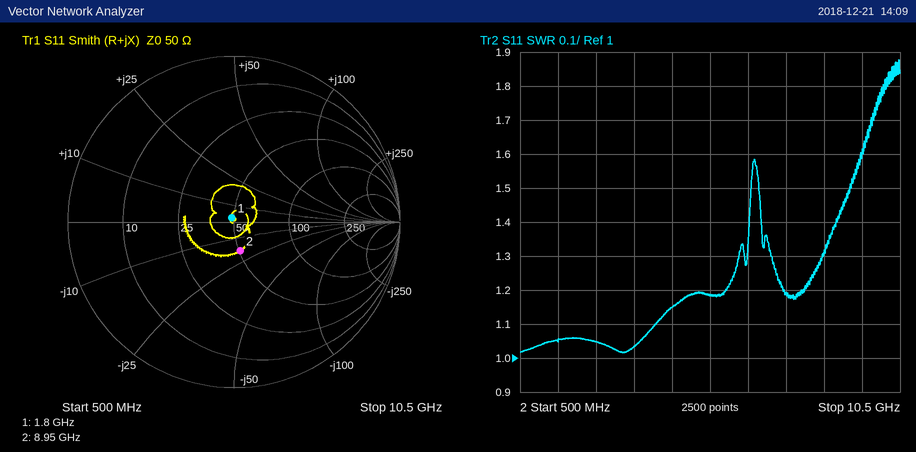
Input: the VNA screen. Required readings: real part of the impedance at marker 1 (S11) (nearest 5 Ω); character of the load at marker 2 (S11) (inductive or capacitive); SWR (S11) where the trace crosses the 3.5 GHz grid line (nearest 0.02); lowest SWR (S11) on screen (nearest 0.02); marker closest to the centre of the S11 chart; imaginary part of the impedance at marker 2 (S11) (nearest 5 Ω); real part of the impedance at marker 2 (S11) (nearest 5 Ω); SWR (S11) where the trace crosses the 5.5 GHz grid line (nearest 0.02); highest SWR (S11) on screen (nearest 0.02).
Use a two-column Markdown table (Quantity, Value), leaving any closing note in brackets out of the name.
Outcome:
| Quantity | Value |
|---|---|
| real part of the impedance at marker 1 (S11) | 50 Ω |
| character of the load at marker 2 (S11) | capacitive |
| SWR (S11) where the trace crosses the 3.5 GHz grid line | 1.04 |
| lowest SWR (S11) on screen | 1.02 |
| marker closest to the centre of the S11 chart | marker 1 |
| imaginary part of the impedance at marker 2 (S11) | -20 Ω |
| real part of the impedance at marker 2 (S11) | 50 Ω |
| SWR (S11) where the trace crosses the 5.5 GHz grid line | 1.18 |
| highest SWR (S11) on screen | 1.88 |
